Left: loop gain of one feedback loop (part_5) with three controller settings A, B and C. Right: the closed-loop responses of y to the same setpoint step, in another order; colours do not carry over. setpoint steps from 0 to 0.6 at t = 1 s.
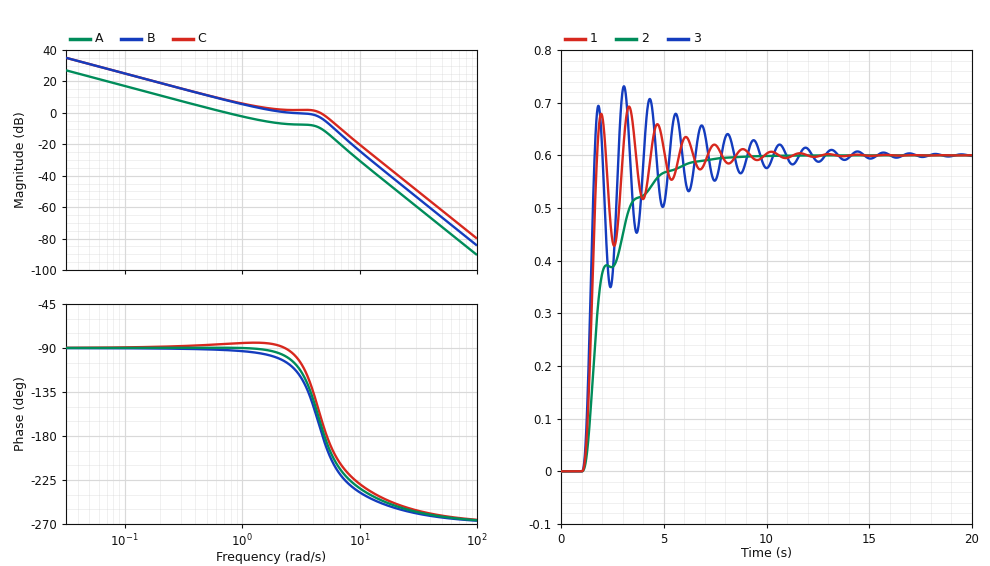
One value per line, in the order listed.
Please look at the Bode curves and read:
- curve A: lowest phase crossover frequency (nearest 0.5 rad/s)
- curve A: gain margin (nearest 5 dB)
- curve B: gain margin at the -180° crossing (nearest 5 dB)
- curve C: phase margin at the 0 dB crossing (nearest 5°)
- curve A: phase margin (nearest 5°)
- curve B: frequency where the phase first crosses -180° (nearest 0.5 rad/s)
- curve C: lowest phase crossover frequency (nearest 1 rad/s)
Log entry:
5.0 rad/s
10 dB
5 dB
20°
90°
5.0 rad/s
5 rad/s
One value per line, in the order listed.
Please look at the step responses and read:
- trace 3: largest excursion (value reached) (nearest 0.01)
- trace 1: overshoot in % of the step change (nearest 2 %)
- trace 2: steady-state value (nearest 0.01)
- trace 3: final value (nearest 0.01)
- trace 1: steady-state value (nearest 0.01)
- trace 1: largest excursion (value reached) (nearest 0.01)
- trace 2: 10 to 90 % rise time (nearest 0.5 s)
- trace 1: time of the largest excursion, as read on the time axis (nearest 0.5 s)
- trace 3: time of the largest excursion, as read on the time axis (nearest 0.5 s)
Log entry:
0.73
16 %
0.60
0.60
0.60
0.69
3.0 s
3.5 s
3.0 s
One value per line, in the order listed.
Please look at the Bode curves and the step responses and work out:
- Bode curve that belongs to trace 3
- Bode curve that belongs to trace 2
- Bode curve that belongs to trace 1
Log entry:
C
A
B
